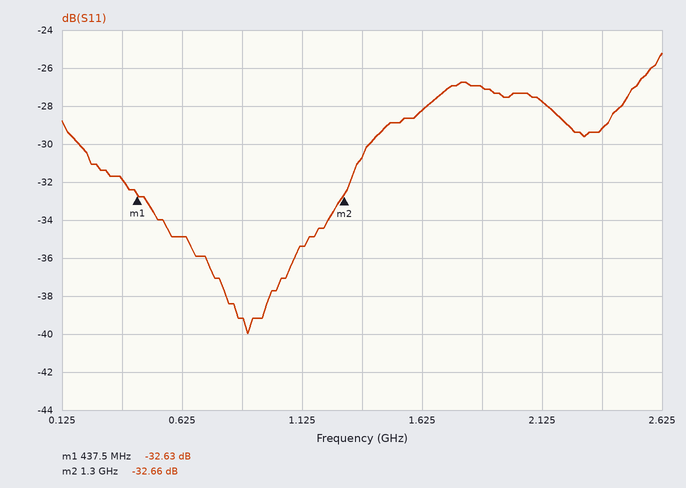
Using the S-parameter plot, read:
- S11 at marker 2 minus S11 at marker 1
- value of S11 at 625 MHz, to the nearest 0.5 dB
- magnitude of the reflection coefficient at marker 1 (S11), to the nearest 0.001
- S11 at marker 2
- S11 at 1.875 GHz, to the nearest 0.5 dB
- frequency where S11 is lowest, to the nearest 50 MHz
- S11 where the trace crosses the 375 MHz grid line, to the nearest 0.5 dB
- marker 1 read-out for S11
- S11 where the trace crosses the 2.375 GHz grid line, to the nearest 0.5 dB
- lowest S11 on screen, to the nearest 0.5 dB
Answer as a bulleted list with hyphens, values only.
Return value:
- -0.03 dB
- -35.0 dB
- 0.023
- -32.66 dB
- -27.0 dB
- 900 MHz
- -32.0 dB
- -32.63 dB
- -29.0 dB
- -40.0 dB
